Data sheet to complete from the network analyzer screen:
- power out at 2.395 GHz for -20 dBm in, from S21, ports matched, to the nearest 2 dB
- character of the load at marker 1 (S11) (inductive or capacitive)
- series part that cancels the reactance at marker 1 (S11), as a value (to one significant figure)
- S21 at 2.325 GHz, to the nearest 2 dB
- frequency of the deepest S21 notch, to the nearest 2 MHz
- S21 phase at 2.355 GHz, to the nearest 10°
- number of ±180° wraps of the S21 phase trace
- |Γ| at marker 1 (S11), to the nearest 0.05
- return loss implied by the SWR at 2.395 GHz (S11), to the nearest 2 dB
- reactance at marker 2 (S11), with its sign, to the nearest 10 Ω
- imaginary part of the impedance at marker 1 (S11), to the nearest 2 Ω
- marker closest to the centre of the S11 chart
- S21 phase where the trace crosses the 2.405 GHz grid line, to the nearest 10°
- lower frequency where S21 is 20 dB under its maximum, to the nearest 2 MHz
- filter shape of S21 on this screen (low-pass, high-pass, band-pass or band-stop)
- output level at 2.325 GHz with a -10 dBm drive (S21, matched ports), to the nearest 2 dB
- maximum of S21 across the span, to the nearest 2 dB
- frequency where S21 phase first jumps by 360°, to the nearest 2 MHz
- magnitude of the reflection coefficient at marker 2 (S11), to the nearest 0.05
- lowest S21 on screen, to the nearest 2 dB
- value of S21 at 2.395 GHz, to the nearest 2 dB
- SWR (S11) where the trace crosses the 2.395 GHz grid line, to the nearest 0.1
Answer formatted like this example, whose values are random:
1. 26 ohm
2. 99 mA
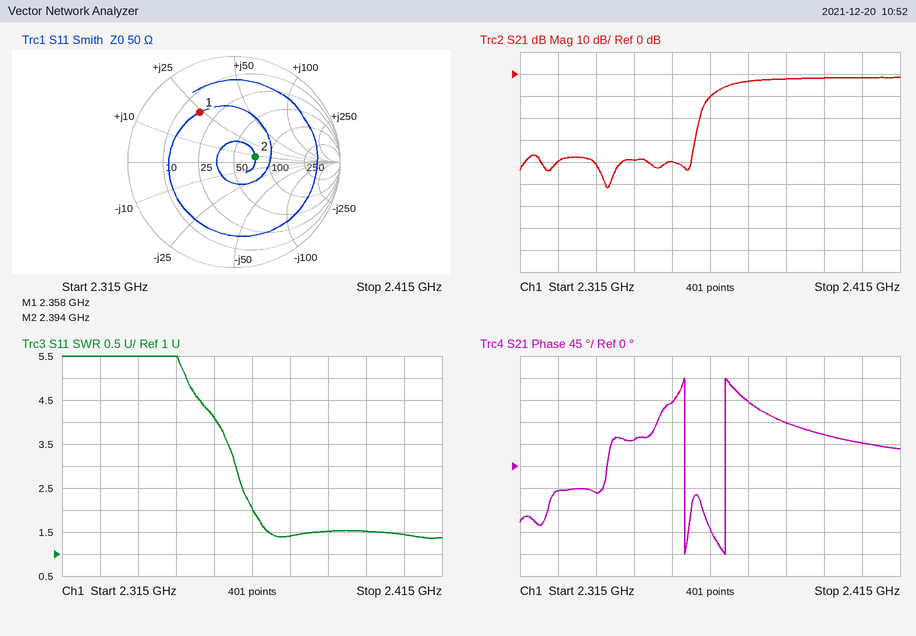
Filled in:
1. -22 dBm
2. inductive
3. 3 pF
4. -40 dB
5. 2.338 GHz
6. 130°
7. 2
8. 0.55
9. 14 dB
10. +10 Ω
11. +24 Ω
12. marker 2
13. 50°
14. 2.362 GHz
15. high-pass
16. -50 dBm
17. -2 dB
18. 2.358 GHz
19. 0.20
20. -52 dB
21. -2 dB
22. 1.5
